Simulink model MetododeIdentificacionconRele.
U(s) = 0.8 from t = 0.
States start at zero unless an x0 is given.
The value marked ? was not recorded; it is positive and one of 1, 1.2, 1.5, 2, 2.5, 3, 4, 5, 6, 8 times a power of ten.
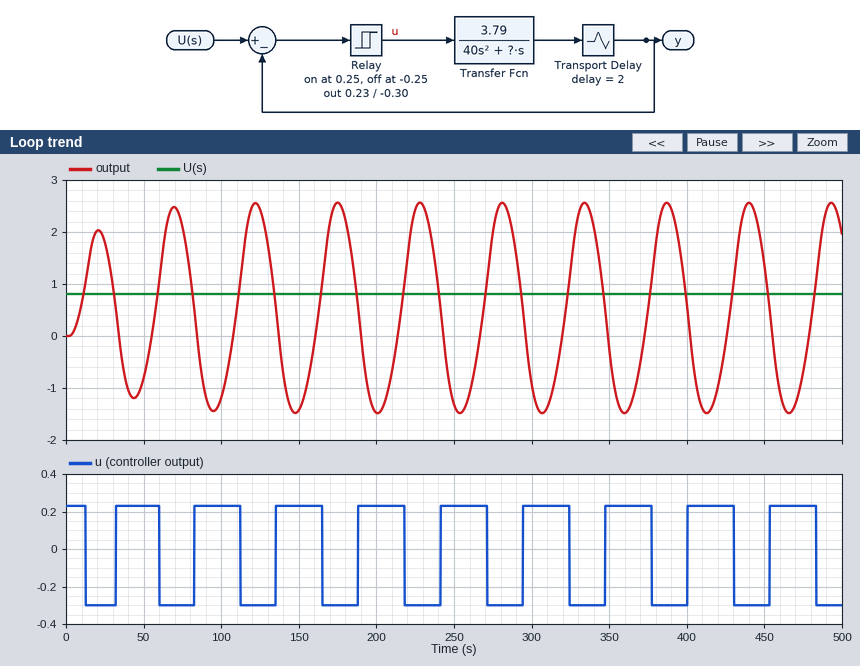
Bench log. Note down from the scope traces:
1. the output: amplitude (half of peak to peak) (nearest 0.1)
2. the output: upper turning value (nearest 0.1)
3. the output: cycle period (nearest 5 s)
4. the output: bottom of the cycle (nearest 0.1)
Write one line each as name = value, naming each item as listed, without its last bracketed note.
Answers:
the output: amplitude (half of peak to peak) = 2.0
the output: upper turning value = 2.6
the output: cycle period = 55 s
the output: bottom of the cycle = -1.5
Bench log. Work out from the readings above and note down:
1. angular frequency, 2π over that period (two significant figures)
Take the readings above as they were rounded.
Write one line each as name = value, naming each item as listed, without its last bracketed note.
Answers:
angular frequency, 2π over that period = 0.11 rad/s
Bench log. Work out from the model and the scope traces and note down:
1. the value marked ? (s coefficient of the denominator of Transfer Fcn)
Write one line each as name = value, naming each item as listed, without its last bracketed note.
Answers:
the value marked ? = 2
